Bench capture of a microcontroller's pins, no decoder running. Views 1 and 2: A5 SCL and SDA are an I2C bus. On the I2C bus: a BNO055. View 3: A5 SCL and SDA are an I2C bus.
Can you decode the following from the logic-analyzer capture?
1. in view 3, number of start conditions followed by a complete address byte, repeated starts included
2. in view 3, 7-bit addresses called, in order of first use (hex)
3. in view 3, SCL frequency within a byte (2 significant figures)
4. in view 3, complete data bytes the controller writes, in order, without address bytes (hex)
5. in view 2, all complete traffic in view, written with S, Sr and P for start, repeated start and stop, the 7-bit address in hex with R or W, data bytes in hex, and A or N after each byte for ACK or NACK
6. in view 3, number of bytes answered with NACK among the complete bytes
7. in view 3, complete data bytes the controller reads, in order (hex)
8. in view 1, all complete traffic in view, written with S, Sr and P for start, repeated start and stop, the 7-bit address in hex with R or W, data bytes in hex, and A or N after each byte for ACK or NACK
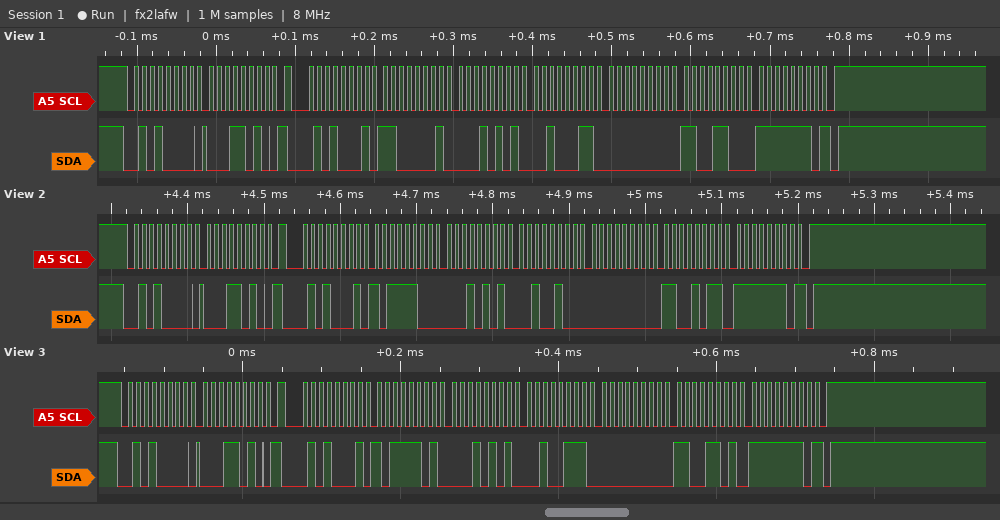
2
0x28
100 kHz
1A
S 28W A 1A A Sr 28R A BC A 15 A 24 A 00 A CB A FE N P
1
BD 15 27 00 CD FE
S 28W A 1A A Sr 28R A C1 A 15 A 23 A 00 A CC A FE N P
